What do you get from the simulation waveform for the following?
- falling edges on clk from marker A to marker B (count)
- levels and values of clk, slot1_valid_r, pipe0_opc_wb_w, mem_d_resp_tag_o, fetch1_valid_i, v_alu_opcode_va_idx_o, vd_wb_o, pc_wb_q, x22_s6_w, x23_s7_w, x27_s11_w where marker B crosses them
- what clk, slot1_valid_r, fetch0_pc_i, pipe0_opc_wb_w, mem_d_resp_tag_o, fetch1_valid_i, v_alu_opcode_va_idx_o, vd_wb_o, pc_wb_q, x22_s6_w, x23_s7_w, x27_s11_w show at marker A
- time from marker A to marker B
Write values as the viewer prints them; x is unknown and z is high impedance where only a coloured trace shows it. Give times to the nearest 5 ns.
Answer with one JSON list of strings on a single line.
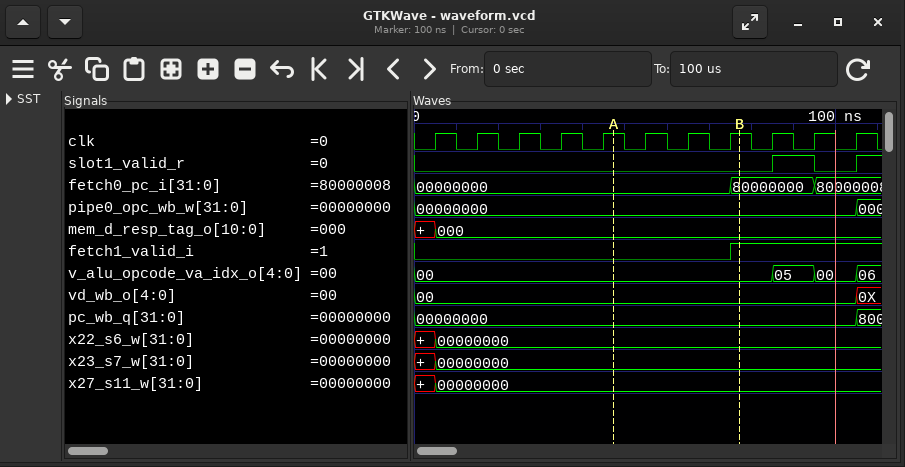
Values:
["3", "clk=1, slot1_valid_r=0, pipe0_opc_wb_w=00000000, mem_d_resp_tag_o=000, fetch1_valid_i=1, v_alu_opcode_va_idx_o=00, vd_wb_o=00, pc_wb_q=00000000, x22_s6_w=00000000, x23_s7_w=00000000, x27_s11_w=00000000", "clk=1, slot1_valid_r=0, fetch0_pc_i=00000000, pipe0_opc_wb_w=00000000, mem_d_resp_tag_o=000, fetch1_valid_i=0, v_alu_opcode_va_idx_o=00, vd_wb_o=00, pc_wb_q=00000000, x22_s6_w=00000000, x23_s7_w=00000000, x27_s11_w=00000000", "30 ns"]
